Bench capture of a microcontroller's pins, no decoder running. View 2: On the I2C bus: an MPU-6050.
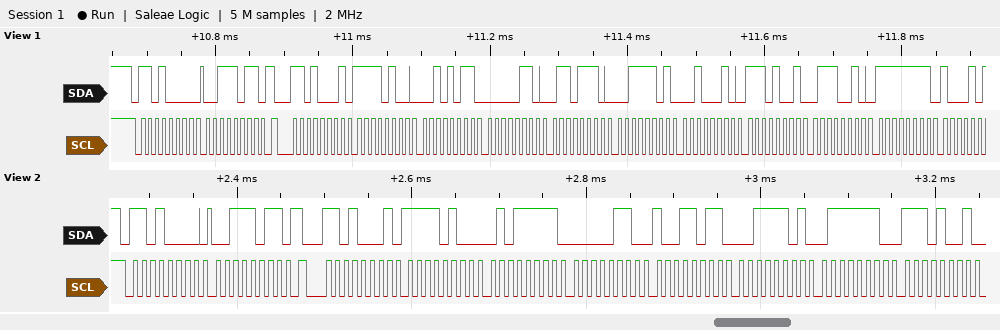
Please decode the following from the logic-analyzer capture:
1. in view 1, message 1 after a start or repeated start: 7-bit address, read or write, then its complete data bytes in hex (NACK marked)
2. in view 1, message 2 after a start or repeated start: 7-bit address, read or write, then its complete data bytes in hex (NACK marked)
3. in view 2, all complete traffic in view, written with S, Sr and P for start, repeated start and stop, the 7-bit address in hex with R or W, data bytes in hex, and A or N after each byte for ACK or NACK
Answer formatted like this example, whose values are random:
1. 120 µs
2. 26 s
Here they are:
1. 0x68 write: 3B
2. 0x68 read: F4 2B 06 6E 3D 22 E9 72 FF
3. S 68W A 3B A Sr 68R A F4 A 5F A 06 A 9B A 3D A 7E A E9 A
